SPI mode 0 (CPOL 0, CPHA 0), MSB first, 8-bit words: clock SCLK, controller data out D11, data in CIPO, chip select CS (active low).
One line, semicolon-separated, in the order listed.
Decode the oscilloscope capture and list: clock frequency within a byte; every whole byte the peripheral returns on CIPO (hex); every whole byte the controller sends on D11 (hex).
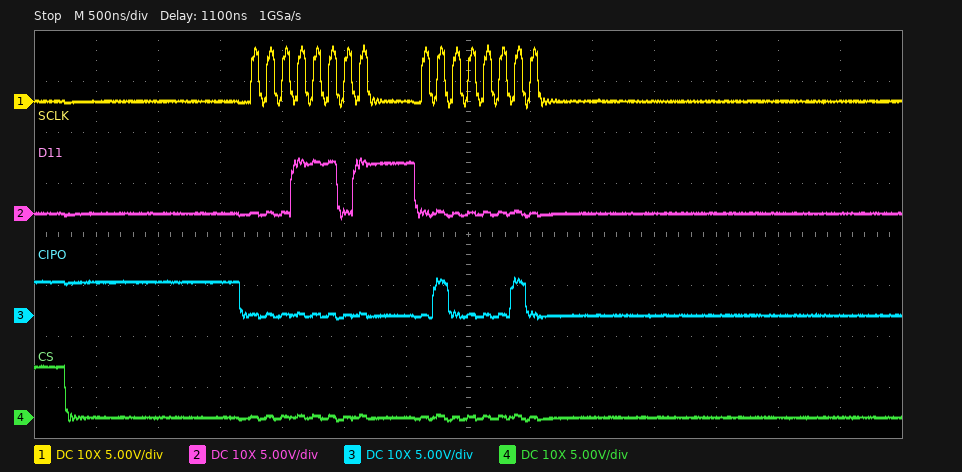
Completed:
8 MHz; 00 42; 1D 00
